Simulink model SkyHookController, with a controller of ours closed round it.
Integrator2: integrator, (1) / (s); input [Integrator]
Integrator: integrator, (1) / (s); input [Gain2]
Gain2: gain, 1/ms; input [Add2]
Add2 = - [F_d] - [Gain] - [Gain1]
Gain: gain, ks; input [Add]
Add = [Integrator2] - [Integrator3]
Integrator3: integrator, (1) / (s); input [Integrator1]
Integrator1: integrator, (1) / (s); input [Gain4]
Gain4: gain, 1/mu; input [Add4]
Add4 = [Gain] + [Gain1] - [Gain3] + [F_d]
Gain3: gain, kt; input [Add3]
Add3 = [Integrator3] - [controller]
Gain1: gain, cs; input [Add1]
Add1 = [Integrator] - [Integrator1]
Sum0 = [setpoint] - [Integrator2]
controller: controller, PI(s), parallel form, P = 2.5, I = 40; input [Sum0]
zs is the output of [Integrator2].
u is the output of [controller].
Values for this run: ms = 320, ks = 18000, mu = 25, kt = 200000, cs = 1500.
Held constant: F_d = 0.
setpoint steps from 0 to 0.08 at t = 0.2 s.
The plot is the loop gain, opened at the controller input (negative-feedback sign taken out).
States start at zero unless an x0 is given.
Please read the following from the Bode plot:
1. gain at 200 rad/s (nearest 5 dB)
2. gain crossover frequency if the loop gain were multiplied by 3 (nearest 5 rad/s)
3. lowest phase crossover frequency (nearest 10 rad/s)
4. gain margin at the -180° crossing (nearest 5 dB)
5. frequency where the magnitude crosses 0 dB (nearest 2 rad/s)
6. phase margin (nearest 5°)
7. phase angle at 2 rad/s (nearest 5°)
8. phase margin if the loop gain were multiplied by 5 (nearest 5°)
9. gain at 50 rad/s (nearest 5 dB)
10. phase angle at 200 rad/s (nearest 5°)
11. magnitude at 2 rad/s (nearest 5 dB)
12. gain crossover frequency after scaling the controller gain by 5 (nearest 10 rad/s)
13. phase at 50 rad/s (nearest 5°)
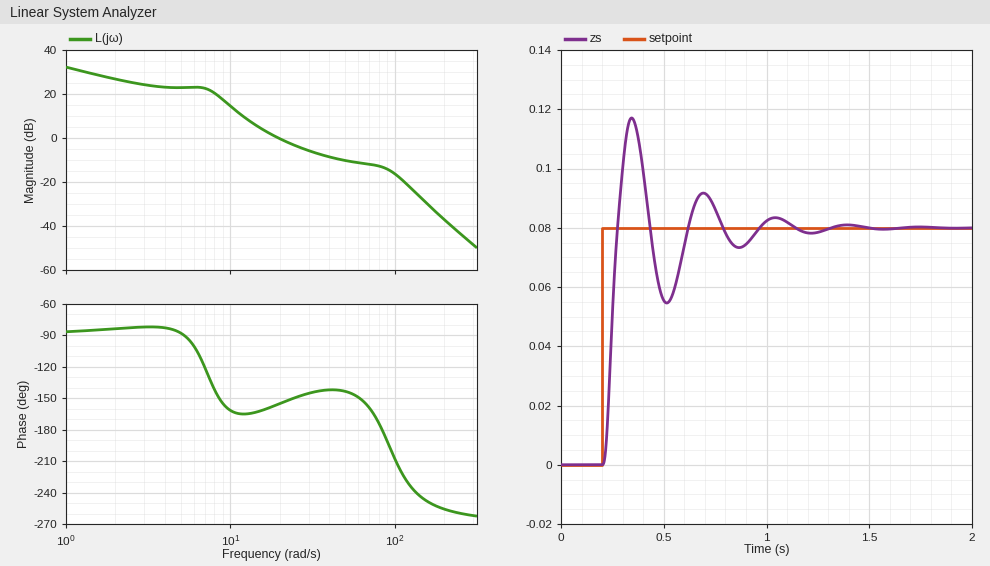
-35 dB
45 rad/s
80 rad/s
15 dB
20 rad/s
25°
-85°
-10°
-10 dB
-255°
25 dB
90 rad/s
-145°
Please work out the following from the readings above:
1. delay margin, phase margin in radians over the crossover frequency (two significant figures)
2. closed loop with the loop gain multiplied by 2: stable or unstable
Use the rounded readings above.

0.022 s
stable
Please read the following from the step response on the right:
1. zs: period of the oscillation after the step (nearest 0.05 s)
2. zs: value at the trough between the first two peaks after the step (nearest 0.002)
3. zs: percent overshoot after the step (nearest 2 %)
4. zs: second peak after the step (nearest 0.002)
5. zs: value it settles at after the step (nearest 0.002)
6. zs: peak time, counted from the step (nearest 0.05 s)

0.35 s
0.054
46 %
0.092
0.080
0.15 s
